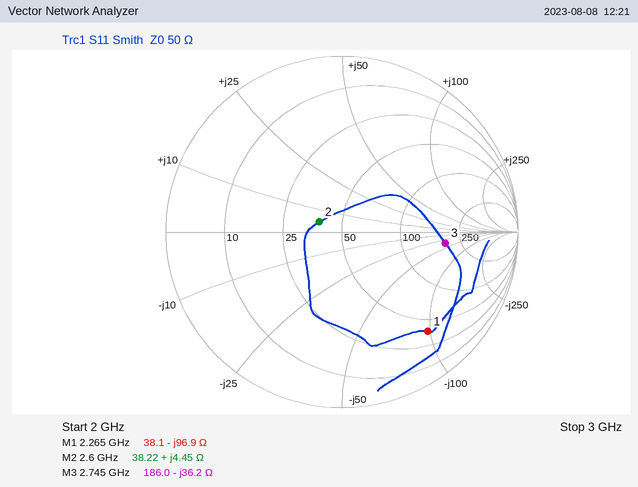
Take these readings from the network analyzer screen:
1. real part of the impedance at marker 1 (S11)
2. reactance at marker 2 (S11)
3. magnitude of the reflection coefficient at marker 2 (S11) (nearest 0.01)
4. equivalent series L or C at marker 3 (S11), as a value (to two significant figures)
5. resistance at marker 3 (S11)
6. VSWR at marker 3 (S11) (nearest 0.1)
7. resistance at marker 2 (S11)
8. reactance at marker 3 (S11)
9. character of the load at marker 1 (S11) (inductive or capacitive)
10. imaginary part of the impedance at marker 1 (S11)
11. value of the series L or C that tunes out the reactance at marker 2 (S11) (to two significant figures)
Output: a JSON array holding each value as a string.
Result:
["38.1 Ω", "+4.45 Ω", "0.14", "1.6 pF", "186.0 Ω", "3.9", "38.22 Ω", "-36.2 Ω", "capacitive", "-96.9 Ω", "14 pF"]
